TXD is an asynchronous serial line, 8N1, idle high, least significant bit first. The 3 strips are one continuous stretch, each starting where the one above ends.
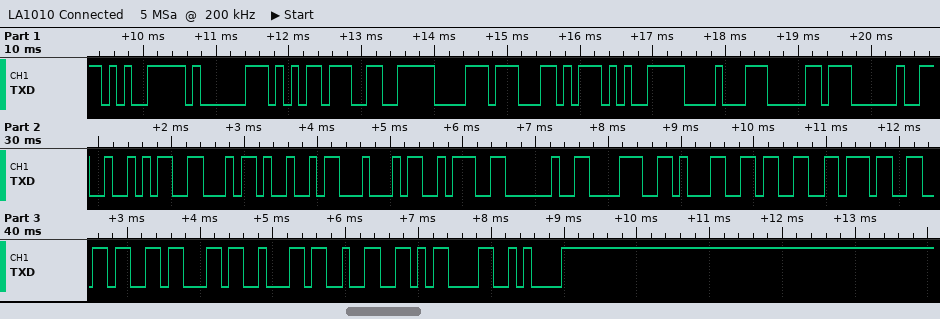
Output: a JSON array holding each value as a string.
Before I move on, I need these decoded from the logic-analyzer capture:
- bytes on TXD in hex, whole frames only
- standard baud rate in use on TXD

["0xE5 0x81 0xB5 0xE6 0xB8 0xAC 0xE5 0x88 0xB0 0x20 0x52 0x46 0x49 0x44 0x3A 0x20 0x38 0x31 0x33 0x37 0x36 0x63 0x62 0x32 0x0D 0x0A", "9600 baud"]
